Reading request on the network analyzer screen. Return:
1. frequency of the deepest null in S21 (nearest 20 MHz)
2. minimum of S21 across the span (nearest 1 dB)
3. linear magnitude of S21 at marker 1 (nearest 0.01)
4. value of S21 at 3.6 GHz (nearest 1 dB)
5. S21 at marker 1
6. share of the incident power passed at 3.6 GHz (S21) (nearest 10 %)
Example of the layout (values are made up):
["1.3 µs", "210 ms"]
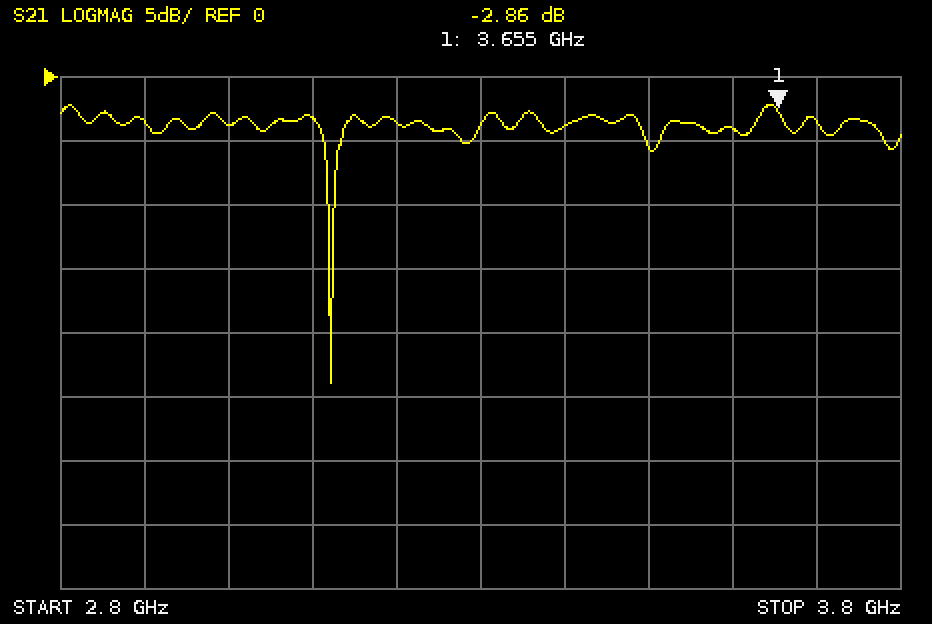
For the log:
["3.12 GHz", "-24 dB", "0.72", "-4 dB", "-2.86 dB", "40 %"]
